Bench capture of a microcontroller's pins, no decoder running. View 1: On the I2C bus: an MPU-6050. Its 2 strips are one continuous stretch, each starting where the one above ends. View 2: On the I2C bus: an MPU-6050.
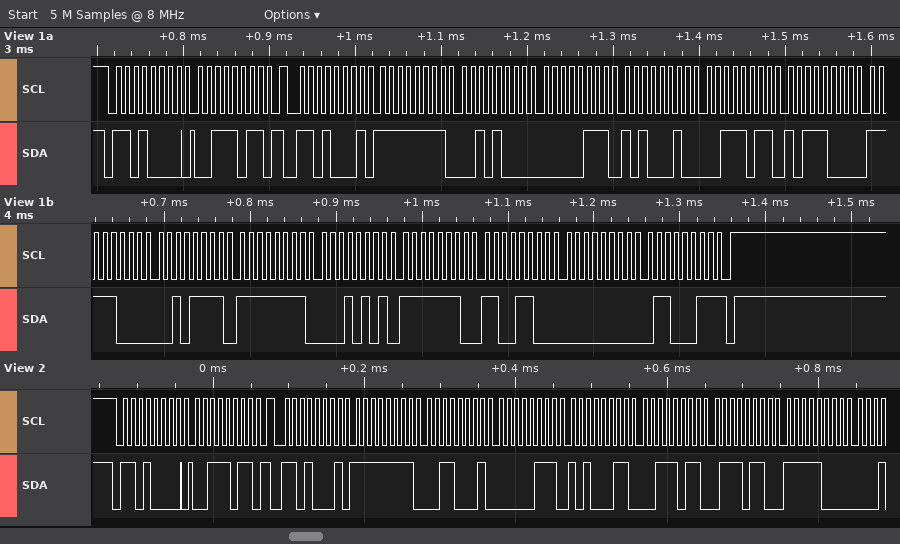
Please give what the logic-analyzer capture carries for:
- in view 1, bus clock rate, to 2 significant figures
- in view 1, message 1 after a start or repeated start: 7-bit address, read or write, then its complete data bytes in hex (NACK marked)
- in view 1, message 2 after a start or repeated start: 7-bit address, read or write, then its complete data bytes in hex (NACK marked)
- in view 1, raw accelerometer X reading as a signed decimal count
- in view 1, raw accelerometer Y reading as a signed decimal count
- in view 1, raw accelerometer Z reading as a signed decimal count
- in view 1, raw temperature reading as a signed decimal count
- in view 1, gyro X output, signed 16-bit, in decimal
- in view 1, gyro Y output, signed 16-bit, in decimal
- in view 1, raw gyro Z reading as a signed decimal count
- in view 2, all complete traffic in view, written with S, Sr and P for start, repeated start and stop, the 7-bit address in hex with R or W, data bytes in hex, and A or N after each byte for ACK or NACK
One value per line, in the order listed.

100 kHz
0x68 write: 3B
0x68 read: FF 28 07 A2 3B B8 F8 2F FF 15 FE CC 00 63 NACK
-216
1954
15288
-2001
-235
-308
99
S 68W A 3B A Sr 68R A FF A 31 A 07 A A3 A 3B A 76 A F8 A
